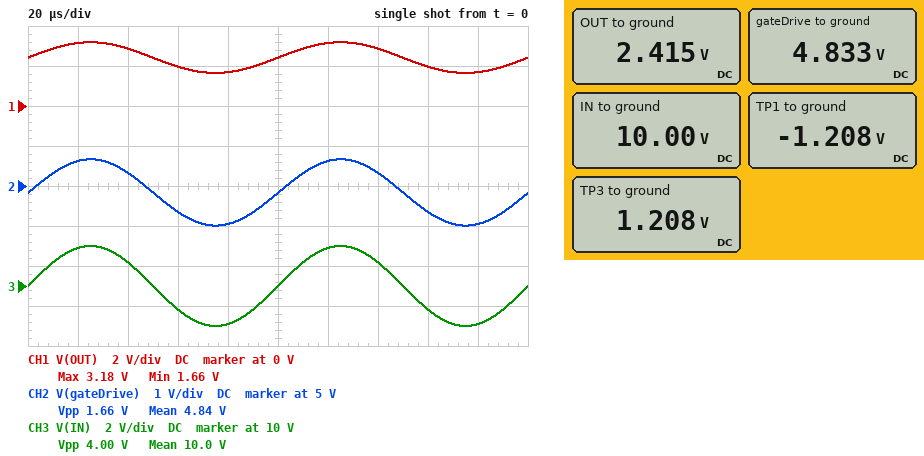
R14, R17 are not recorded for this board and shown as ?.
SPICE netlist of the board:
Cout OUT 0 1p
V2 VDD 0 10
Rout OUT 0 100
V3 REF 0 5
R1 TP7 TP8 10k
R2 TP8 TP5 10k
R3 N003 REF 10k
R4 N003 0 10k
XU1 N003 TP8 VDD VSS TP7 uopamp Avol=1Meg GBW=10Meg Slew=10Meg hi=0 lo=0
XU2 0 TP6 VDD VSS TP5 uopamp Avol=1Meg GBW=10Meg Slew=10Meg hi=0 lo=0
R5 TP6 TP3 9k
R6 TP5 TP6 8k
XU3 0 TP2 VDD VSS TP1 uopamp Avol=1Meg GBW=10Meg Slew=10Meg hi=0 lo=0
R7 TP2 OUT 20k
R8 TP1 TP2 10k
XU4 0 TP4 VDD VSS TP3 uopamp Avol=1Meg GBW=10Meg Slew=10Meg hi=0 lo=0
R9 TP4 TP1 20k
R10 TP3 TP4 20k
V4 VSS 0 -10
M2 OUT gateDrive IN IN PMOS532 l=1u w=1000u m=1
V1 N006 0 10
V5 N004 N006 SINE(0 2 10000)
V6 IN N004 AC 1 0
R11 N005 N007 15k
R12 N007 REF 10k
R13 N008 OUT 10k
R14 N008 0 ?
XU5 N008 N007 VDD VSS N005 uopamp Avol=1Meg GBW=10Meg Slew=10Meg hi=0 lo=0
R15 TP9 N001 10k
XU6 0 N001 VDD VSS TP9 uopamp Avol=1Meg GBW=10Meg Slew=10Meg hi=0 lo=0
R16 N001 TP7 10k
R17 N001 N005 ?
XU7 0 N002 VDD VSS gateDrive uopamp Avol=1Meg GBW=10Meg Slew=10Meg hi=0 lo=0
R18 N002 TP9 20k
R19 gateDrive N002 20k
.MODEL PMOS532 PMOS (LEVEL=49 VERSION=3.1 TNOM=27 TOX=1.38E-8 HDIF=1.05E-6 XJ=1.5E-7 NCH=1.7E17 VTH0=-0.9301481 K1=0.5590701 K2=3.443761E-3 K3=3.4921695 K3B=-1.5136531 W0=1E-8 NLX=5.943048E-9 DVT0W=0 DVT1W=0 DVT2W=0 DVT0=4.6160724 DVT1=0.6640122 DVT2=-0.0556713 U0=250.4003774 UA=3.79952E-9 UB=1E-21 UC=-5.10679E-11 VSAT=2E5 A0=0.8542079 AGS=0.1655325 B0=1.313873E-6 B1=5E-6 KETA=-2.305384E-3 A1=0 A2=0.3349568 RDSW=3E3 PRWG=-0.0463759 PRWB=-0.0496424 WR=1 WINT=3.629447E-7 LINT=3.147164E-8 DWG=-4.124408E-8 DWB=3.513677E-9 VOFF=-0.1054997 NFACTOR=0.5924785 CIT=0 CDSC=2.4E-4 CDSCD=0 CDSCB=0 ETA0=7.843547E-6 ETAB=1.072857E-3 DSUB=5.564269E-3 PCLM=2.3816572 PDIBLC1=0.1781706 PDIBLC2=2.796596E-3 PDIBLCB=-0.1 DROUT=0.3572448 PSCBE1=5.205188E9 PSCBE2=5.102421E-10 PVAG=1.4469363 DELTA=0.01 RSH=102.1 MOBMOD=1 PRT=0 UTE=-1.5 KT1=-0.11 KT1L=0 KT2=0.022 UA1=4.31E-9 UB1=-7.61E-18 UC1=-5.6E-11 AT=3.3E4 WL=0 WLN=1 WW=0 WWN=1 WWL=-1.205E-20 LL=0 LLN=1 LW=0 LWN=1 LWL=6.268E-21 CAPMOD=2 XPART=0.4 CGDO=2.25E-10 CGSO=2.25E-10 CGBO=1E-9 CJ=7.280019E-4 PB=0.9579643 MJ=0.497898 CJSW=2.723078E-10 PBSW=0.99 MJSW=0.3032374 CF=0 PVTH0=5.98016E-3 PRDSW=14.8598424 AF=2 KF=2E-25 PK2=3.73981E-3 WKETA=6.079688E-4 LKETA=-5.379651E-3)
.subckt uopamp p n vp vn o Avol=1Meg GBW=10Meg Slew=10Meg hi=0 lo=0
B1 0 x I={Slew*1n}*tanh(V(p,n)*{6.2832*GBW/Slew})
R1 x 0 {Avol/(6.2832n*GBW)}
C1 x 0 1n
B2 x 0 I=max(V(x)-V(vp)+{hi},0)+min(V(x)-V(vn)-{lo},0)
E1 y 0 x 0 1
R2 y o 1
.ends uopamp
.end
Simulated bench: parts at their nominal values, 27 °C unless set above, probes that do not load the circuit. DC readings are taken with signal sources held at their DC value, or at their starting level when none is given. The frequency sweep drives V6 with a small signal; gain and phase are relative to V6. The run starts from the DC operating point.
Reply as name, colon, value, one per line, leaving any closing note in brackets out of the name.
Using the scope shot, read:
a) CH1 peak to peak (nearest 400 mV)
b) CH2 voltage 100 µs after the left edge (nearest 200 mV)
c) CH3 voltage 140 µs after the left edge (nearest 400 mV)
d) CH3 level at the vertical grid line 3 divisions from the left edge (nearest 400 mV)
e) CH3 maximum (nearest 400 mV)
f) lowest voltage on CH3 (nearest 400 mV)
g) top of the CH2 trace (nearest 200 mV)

CH1 peak to peak: 1.6 V
CH2 voltage 100 µs after the left edge: 4.8 V
CH3 voltage 140 µs after the left edge: 11.2 V
CH3 level at the vertical grid line 3 divisions from the left edge: 8.8 V
CH3 maximum: 12.0 V
lowest voltage on CH3: 8.0 V
top of the CH2 trace: 5.6 V
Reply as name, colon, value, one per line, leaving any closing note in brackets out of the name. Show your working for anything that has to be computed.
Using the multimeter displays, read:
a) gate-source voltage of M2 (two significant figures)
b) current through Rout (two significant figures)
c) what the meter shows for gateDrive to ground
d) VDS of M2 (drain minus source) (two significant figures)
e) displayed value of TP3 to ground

gate-source voltage of M2: 4.833 V - 10 V = -5.2 V
current through Rout: (2.415 V) / 100 Ω = 24 mA
what the meter shows for gateDrive to ground: 4.833 V
VDS of M2 (drain minus source): 2.415 V - 10 V = -7.6 V
displayed value of TP3 to ground: 1.208 V
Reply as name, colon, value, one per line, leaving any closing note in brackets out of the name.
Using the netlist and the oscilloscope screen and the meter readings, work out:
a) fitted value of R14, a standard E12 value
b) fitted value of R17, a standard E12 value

fitted value of R14, a standard E12 value: 22 kΩ
fitted value of R17, a standard E12 value: 27 kΩ
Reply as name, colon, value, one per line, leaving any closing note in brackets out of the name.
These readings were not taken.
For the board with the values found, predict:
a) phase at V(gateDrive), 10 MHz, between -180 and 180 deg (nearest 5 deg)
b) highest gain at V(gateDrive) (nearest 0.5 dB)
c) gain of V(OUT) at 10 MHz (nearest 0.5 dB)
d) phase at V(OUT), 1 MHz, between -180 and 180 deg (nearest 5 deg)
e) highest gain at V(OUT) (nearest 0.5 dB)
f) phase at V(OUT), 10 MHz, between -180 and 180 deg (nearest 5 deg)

phase at V(gateDrive), 10 MHz, between -180 and 180 deg: 160 deg
highest gain at V(gateDrive): -7.5 dB
gain of V(OUT) at 10 MHz: -3.5 dB
phase at V(OUT), 1 MHz, between -180 and 180 deg: 20 deg
highest gain at V(OUT): -2.5 dB
phase at V(OUT), 10 MHz, between -180 and 180 deg: 0 deg
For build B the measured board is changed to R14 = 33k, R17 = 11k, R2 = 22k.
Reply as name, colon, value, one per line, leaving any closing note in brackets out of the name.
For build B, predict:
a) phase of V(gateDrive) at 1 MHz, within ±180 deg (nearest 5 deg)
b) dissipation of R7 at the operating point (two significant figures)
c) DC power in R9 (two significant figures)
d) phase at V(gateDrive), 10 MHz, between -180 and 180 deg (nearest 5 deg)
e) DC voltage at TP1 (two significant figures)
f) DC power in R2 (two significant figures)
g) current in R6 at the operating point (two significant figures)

phase of V(gateDrive) at 1 MHz, within ±180 deg: -40 deg
dissipation of R7 at the operating point: 470 µW
DC power in R9: 120 µW
phase at V(gateDrive), 10 MHz, between -180 and 180 deg: 155 deg
DC voltage at TP1: -1.5 V
DC power in R2: 680 µW
current in R6 at the operating point: 170 µA
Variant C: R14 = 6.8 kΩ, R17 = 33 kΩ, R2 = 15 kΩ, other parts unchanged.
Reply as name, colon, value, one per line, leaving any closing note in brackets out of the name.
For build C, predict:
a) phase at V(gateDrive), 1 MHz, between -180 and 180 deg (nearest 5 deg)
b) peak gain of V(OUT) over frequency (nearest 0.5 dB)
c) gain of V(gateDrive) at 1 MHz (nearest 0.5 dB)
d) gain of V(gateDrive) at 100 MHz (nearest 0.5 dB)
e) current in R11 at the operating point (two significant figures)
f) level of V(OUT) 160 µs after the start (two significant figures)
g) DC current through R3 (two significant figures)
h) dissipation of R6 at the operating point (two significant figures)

phase at V(gateDrive), 1 MHz, between -180 and 180 deg: -45 deg
peak gain of V(OUT) over frequency: -7.5 dB
gain of V(gateDrive) at 1 MHz: -14.0 dB
gain of V(gateDrive) at 100 MHz: -59.5 dB
current in R11 at the operating point: 380 µA
level of V(OUT) 160 µs after the start: 2.5 V
DC current through R3: 250 µA
dissipation of R6 at the operating point: 220 µW
